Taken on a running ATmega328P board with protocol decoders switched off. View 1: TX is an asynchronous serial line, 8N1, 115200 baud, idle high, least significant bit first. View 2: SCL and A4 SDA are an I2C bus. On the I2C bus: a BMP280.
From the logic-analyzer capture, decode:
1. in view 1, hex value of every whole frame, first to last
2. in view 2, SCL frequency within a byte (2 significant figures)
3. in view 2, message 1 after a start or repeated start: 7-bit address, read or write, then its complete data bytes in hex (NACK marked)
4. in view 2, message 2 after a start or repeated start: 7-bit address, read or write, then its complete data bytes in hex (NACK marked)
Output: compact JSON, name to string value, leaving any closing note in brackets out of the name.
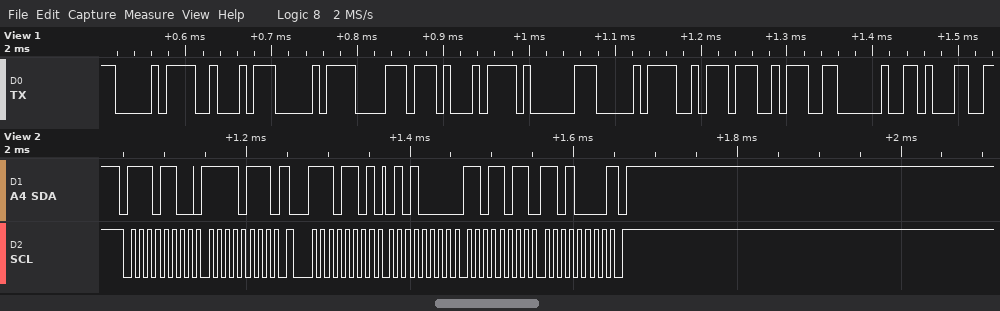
{"in view 1, hex value of every whole frame, first to last": "D0 A2 D0 B8 D1 81 D0 BA 3A 20 31", "in view 2, SCL frequency within a byte": "100 kHz", "in view 2, message 1 after a start or repeated start: 7-bit address, read or write, then its complete data bytes in hex": "0x76 write: F7", "in view 2, message 2 after a start or repeated start: 7-bit address, read or write, then its complete data bytes in hex": "0x76 read: 50 DB D0 NACK"}
